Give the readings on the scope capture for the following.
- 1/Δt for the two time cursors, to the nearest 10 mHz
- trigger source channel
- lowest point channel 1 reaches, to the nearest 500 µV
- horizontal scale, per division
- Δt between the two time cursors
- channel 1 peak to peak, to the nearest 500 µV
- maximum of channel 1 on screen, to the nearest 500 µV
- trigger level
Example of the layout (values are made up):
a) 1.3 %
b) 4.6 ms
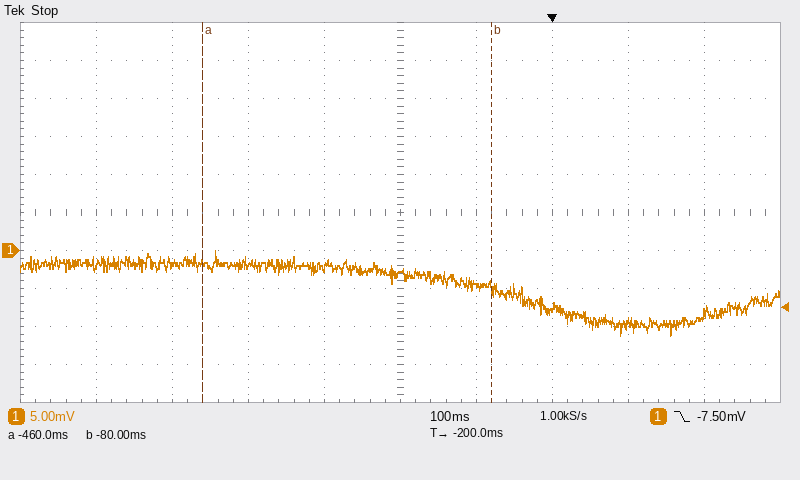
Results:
a) 2.63 Hz
b) channel 1
c) -11.0 mV
d) 100 ms
e) 380 ms
f) 11.0 mV
g) 0.0 mV
h) -7.50 mV
